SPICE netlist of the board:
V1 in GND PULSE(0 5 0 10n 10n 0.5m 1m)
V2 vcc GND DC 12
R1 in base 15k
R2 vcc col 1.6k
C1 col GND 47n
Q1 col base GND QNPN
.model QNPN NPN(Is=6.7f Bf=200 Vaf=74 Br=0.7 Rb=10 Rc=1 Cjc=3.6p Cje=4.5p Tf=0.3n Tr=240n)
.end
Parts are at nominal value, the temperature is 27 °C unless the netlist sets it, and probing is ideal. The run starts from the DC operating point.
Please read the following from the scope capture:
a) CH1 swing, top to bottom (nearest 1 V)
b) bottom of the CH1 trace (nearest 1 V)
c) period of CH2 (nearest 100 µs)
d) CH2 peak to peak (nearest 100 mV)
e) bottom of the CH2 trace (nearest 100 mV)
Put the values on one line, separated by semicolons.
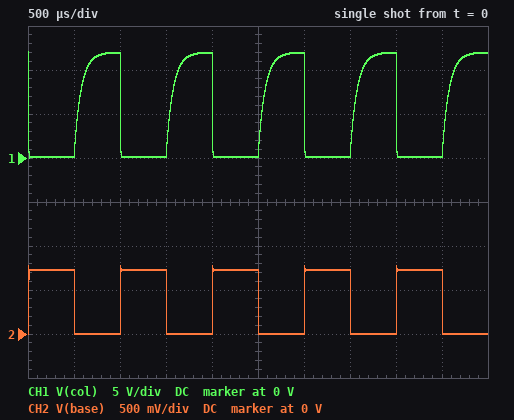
12 V; 0 V; 1.0 ms; 800 mV; 0 V
